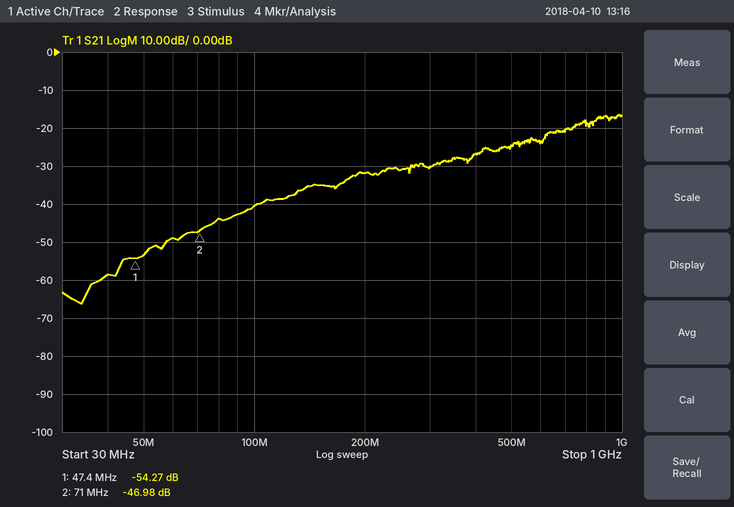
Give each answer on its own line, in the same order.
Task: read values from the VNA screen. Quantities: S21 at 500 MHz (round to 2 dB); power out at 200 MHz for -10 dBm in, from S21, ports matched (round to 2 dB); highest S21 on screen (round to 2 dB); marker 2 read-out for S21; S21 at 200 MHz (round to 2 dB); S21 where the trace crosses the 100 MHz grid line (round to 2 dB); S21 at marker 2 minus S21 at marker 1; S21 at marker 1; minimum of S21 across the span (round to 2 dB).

-24 dB
-42 dBm
-16 dB
-46.98 dB
-32 dB
-40 dB
7.29 dB
-54.27 dB
-66 dB
